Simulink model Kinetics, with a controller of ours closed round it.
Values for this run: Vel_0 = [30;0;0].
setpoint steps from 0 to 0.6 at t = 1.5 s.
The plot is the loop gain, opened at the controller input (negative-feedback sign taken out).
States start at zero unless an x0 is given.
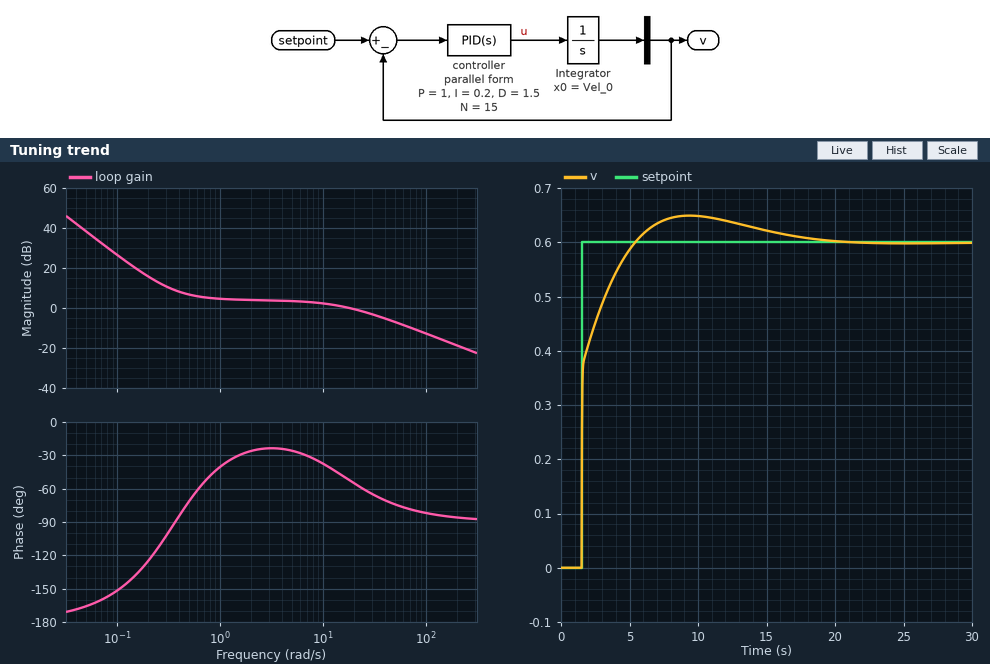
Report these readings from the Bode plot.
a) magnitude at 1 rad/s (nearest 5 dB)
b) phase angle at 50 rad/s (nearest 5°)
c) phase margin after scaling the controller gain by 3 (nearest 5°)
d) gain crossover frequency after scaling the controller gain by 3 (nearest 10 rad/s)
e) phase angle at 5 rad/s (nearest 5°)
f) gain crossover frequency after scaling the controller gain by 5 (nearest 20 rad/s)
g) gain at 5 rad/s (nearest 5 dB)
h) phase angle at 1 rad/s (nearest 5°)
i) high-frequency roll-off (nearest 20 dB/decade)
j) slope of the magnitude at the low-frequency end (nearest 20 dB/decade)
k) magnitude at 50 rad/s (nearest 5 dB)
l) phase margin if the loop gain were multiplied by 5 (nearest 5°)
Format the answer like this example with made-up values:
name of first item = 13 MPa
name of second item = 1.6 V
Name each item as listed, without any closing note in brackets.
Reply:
magnitude at 1 rad/s = 5 dB
phase angle at 50 rad/s = -75°
phase margin after scaling the controller gain by 3 = 100°
gain crossover frequency after scaling the controller gain by 3 = 70 rad/s
phase angle at 5 rad/s = -25°
gain crossover frequency after scaling the controller gain by 5 = 120 rad/s
gain at 5 rad/s = 5 dB
phase angle at 1 rad/s = -40°
high-frequency roll-off = -20 dB/decade
slope of the magnitude at the low-frequency end = -40 dB/decade
magnitude at 50 rad/s = -5 dB
phase margin if the loop gain were multiplied by 5 = 95°
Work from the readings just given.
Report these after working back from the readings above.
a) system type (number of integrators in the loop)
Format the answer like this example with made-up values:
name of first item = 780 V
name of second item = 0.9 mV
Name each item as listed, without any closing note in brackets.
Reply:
system type = 2
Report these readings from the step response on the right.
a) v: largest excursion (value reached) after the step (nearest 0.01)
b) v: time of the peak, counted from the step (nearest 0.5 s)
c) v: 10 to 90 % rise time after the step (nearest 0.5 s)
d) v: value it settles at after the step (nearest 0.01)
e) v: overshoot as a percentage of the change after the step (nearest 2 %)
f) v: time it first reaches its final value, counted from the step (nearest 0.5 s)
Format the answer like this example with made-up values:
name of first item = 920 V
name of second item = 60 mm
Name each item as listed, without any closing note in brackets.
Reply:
v: largest excursion (value reached) after the step = 0.65
v: time of the peak, counted from the step = 8.0 s
v: 10 to 90 % rise time after the step = 2.5 s
v: value it settles at after the step = 0.60
v: overshoot as a percentage of the change after the step = 8 %
v: time it first reaches its final value, counted from the step = 4.0 s
